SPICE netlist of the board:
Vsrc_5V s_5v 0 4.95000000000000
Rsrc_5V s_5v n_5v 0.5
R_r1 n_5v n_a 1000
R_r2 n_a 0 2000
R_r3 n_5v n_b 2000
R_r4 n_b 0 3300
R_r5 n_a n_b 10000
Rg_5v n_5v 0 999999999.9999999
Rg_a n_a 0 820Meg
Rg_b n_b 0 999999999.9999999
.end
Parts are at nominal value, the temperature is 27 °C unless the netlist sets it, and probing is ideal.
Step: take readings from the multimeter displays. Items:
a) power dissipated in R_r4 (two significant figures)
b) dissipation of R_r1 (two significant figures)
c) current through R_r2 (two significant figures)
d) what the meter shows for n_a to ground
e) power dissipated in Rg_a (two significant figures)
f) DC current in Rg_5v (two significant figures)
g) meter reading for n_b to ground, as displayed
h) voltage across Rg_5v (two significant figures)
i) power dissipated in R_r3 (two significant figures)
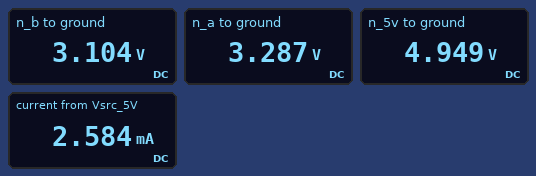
2.9 mW
2.8 mW
1.6 mA
3.287 V
13 nW
4.9 nA
3.104 V
4.9 V
1.7 mW
